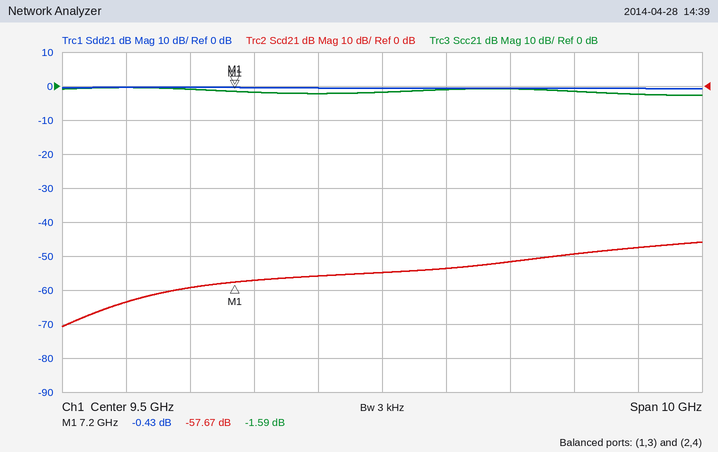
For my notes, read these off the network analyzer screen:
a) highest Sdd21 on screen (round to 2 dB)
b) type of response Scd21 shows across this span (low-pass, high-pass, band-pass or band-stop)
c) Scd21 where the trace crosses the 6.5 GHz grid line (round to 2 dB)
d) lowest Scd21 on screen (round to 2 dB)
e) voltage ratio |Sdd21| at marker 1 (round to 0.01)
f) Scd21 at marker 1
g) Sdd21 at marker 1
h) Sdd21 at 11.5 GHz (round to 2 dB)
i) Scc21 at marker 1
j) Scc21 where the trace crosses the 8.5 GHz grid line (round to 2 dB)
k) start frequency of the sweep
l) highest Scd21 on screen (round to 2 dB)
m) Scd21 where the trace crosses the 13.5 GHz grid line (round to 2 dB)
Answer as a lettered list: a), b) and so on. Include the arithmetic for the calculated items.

a) 0 dB
b) high-pass
c) -60 dB
d) -70 dB
e) 10^(-0.43/20) ≈ 0.95
f) -57.67 dB
g) -0.43 dB
h) 0 dB
i) -1.59 dB
j) -2 dB
k) 4.5 GHz
l) -46 dB
m) -48 dB
